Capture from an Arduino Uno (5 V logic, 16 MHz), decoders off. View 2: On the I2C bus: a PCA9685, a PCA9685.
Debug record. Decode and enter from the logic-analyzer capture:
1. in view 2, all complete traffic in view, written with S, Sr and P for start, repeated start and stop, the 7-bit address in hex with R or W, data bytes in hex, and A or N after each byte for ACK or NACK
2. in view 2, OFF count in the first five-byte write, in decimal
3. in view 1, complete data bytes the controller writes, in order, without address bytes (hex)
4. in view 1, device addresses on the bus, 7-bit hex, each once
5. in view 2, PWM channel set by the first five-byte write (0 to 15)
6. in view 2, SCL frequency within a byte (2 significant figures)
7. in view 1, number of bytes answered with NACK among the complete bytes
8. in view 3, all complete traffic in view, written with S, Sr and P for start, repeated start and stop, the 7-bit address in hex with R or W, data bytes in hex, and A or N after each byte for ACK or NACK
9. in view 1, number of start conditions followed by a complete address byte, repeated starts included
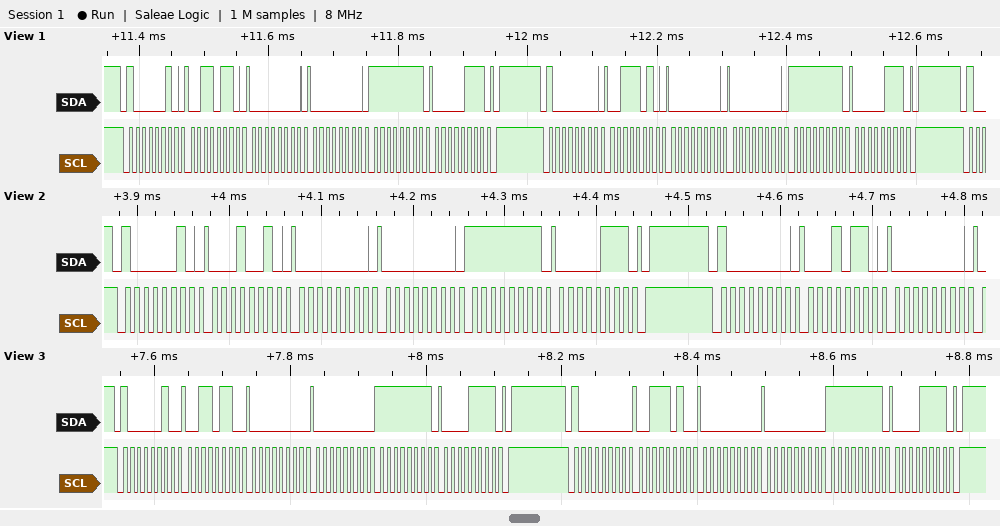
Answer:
S 41W A 12 A 00 A 00 A FF A 07 A P S 40W A 16 A 00 A
2047
36 00 00 FF 07 3A 00 00 FF 07
0x41 0x40
3
100 kHz
0
S 41W A 36 A 00 A 00 A FF A 0F A P S 40W A 3A A 00 A 00 A FF A 0F A P
2
